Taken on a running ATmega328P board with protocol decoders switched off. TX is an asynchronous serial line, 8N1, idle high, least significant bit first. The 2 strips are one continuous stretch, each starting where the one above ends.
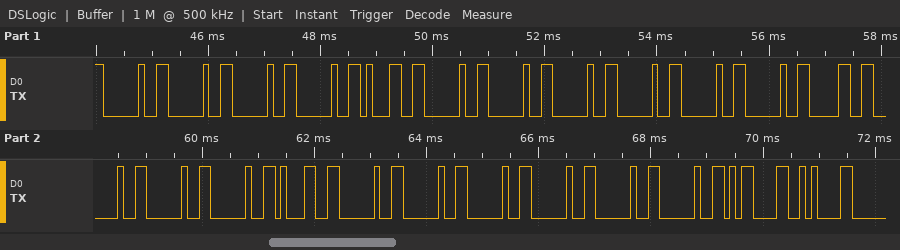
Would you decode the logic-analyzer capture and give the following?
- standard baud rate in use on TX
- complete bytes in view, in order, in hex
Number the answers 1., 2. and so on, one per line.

1. 9600 baud
2. 20 20 20 20 31 20 20 20 20 20 20 30 20 20 20 31 20 20 20 20 20 20 0D 0A
